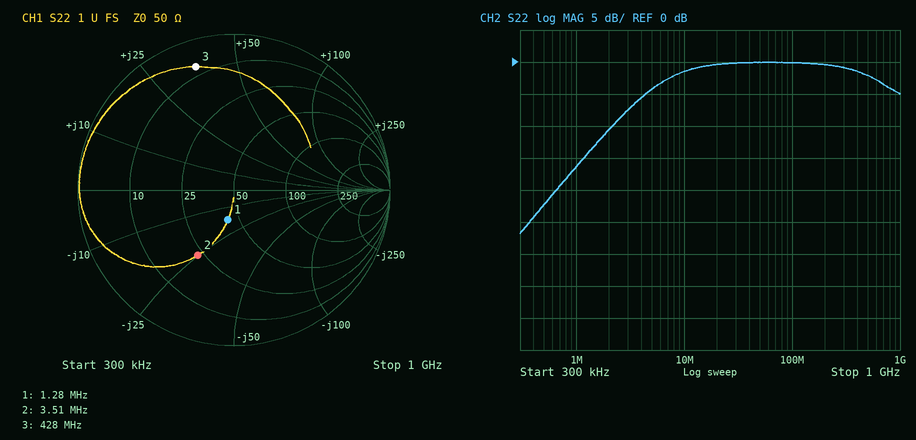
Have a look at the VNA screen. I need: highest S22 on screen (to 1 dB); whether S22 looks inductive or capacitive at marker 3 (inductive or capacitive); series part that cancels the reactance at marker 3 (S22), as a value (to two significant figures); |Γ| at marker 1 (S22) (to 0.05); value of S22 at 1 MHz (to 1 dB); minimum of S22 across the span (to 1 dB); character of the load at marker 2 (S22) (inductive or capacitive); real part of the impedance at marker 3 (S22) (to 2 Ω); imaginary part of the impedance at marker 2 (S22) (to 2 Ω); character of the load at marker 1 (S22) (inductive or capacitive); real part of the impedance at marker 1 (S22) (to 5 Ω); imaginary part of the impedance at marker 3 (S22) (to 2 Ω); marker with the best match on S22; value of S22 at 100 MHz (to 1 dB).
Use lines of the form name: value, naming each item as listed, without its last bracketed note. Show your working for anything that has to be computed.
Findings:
highest S22 on screen: 0 dB
whether S22 looks inductive or capacitive at marker 3: inductive
series part that cancels the reactance at marker 3 (S22), as a value: C = 1/(2π × 428 MHz × 36 Ω) ≈ 10 pF
|Γ| at marker 1 (S22): 0.20
value of S22 at 1 MHz: -16 dB
minimum of S22 across the span: -27 dB
character of the load at marker 2 (S22): capacitive
real part of the impedance at marker 3 (S22): 8 Ω
imaginary part of the impedance at marker 2 (S22): -24 Ω
character of the load at marker 1 (S22): capacitive
real part of the impedance at marker 1 (S22): 45 Ω
imaginary part of the impedance at marker 3 (S22): +36 Ω
marker with the best match on S22: marker 1
value of S22 at 100 MHz: 0 dB
